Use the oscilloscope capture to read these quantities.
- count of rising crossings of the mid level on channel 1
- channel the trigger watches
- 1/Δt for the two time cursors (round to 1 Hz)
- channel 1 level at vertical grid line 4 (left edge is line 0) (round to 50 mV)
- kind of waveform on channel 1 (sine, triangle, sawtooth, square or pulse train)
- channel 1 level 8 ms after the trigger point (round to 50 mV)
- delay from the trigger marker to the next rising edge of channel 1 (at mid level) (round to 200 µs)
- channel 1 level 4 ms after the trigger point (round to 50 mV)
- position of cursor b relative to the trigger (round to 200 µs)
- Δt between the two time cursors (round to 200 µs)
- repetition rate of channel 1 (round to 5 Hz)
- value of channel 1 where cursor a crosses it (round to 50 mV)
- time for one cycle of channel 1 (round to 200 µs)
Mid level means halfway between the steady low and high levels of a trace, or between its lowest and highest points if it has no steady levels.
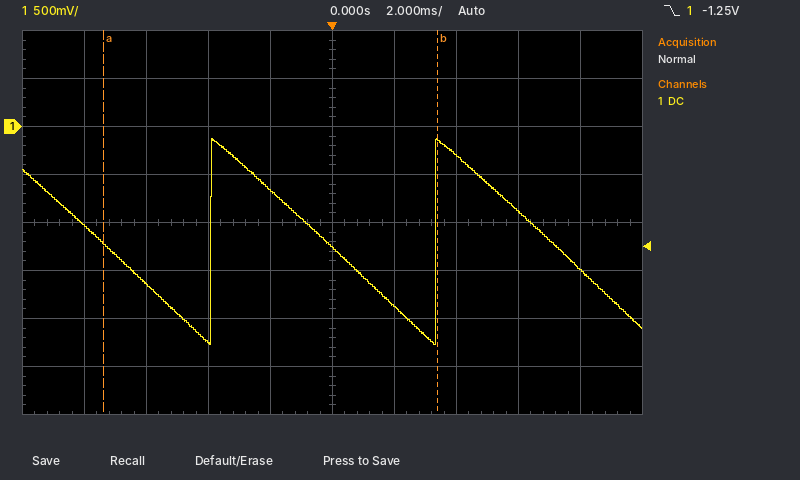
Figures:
2
channel 1
93 Hz
-650 mV
sawtooth
-1.50 V
3.4 ms
-300 mV
+3.4 ms
10.8 ms
140 Hz
-1.20 V
7.2 ms
